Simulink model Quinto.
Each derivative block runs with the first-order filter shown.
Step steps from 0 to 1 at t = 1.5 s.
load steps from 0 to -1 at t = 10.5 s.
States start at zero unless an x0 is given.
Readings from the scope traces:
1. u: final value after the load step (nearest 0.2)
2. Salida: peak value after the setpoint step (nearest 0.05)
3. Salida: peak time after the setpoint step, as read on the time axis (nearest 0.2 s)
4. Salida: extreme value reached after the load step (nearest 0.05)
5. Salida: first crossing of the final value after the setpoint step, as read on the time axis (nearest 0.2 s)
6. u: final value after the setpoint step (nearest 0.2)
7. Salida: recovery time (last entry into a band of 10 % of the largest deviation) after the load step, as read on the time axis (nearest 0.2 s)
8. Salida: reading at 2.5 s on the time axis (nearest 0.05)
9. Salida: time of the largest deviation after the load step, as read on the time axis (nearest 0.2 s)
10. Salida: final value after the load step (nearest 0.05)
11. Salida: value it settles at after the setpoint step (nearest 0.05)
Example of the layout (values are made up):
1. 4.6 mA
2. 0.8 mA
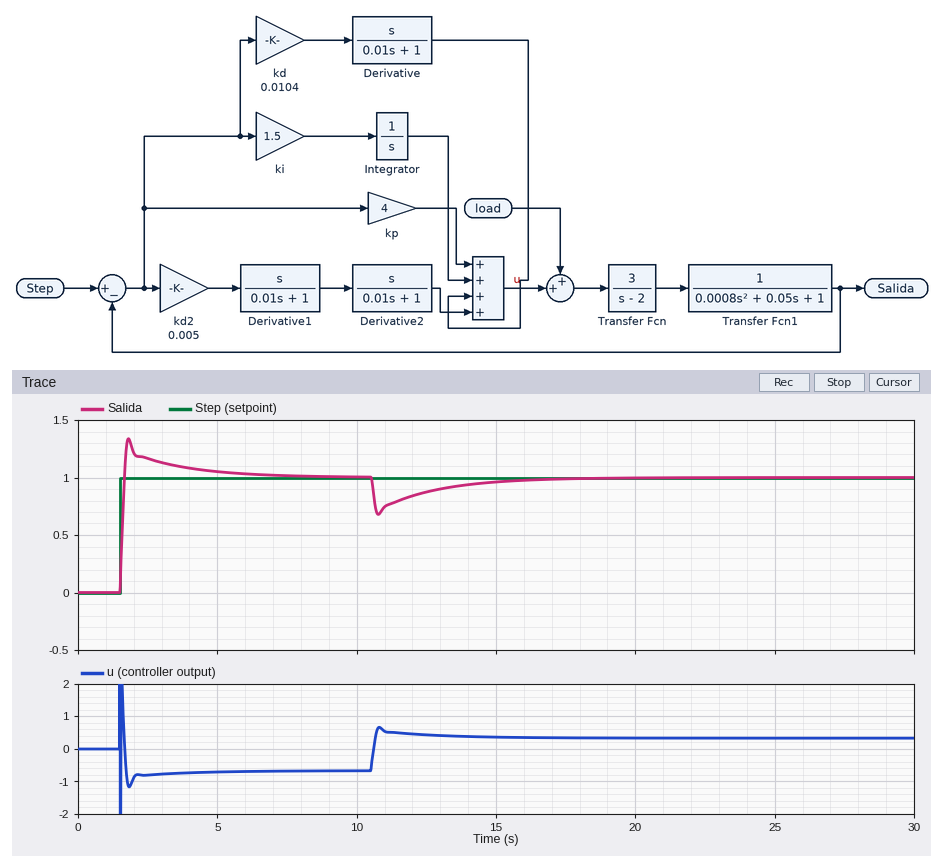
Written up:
1. 0.4
2. 1.35
3. 1.8 s
4. 0.70
5. 1.6 s
6. -0.6
7. 15.4 s
8. 1.15
9. 10.8 s
10. 1.00
11. 1.00
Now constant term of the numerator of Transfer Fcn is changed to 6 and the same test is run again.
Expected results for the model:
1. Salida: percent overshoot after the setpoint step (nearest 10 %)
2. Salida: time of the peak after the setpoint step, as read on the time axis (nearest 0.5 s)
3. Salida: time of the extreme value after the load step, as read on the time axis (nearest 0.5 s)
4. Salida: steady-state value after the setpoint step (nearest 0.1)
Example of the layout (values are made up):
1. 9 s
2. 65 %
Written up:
1. 30 %
2. 1.5 s
3. 10.5 s
4. 1.0
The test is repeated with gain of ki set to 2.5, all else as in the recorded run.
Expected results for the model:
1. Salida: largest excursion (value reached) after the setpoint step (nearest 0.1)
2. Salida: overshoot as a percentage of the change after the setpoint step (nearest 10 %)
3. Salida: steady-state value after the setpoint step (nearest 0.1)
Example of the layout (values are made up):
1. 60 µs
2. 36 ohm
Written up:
1. 1.4
2. 40 %
3. 1.0
